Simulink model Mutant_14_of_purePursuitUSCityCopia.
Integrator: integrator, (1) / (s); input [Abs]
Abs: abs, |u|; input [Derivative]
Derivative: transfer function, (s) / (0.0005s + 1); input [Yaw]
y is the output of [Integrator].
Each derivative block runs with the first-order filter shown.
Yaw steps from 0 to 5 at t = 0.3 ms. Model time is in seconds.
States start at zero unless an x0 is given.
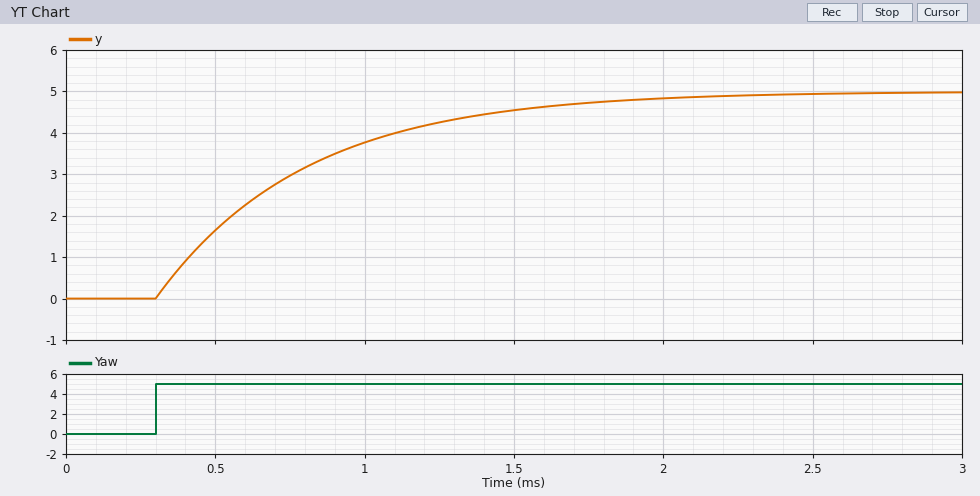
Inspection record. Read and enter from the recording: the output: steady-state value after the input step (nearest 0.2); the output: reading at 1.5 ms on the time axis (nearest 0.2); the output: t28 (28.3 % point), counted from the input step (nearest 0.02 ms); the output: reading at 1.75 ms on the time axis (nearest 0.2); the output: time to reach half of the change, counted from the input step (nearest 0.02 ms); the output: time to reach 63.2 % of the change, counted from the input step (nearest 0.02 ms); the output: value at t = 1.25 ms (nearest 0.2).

5.0
4.6
0.16 ms
4.8
0.34 ms
0.50 ms
4.2
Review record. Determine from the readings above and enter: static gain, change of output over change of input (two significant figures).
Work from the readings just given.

1.0
